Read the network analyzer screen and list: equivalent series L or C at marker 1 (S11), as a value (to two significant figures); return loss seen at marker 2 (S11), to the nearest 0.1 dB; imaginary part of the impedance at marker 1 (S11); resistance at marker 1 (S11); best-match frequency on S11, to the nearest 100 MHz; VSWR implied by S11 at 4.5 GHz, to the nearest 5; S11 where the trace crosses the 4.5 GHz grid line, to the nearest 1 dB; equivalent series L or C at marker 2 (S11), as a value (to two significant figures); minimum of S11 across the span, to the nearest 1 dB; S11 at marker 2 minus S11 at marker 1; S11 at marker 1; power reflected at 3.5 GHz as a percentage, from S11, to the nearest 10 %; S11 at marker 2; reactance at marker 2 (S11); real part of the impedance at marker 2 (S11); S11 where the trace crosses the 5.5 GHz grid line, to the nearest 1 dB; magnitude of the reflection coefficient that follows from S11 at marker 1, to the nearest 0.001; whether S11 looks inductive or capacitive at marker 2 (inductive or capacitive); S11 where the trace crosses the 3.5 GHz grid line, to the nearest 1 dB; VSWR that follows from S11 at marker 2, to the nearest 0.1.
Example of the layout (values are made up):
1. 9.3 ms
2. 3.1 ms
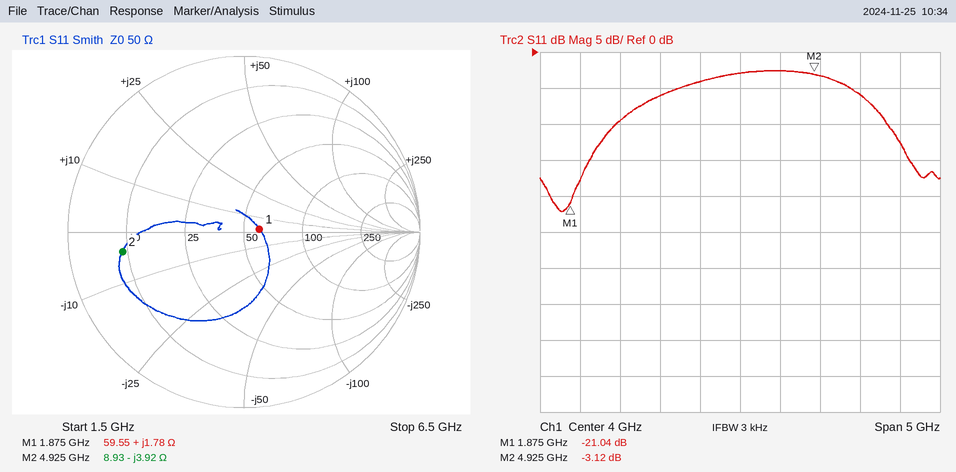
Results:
1. 150 pH
2. 3.1 dB
3. +1.78 Ω
4. 59.55 Ω
5. 1.8 GHz
6. 5
7. -3 dB
8. 8.2 pF
9. -22 dB
10. 17.92 dB
11. -21.04 dB
12. 40 %
13. -3.12 dB
14. -3.92 Ω
15. 8.93 Ω
16. -6 dB
17. 0.089
18. capacitive
19. -4 dB
20. 5.6
